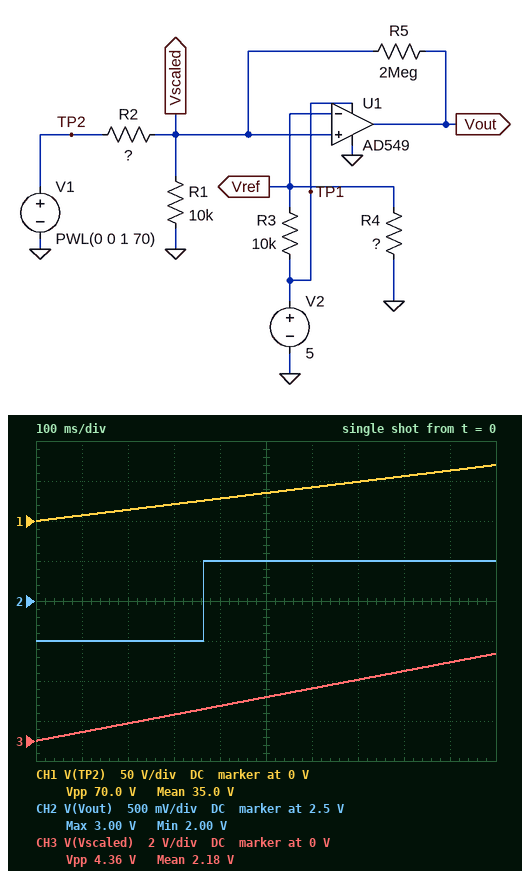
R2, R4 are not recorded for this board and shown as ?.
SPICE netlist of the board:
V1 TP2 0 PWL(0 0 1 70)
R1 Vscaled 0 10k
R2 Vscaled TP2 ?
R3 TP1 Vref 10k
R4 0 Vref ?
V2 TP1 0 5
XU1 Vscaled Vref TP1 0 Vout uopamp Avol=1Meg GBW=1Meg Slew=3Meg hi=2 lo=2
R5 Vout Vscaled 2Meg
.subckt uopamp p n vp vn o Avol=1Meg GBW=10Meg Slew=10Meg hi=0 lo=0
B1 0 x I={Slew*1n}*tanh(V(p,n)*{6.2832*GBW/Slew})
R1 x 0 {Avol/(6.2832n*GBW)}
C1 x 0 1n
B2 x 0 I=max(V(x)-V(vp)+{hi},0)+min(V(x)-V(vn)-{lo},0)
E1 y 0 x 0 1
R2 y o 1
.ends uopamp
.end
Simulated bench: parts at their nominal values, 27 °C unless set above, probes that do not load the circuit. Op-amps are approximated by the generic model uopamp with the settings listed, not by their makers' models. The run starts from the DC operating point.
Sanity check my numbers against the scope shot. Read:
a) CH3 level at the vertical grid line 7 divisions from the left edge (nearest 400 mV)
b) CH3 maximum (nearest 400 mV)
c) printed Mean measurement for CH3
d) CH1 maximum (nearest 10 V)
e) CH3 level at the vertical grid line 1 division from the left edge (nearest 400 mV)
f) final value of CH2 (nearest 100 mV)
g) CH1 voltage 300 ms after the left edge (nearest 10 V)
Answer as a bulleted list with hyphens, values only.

- 3.2 V
- 4.4 V
- 2.18 V
- 70 V
- 400 mV
- 3.0 V
- 20 V
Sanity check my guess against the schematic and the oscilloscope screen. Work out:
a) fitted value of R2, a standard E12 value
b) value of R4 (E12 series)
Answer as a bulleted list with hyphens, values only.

- 150 kΩ
- 4.7 kΩ
